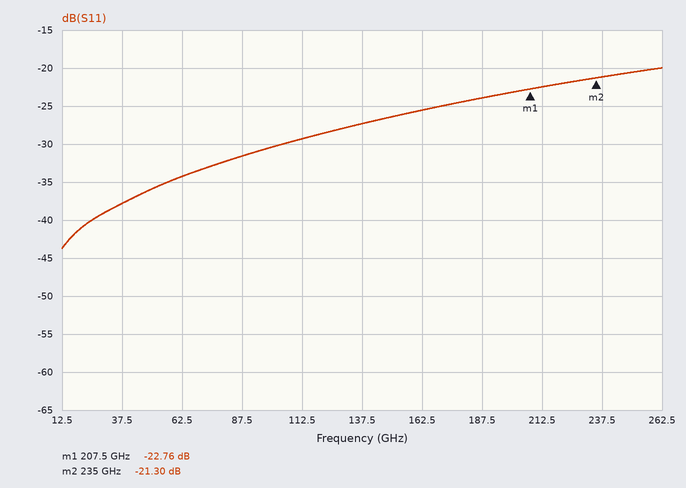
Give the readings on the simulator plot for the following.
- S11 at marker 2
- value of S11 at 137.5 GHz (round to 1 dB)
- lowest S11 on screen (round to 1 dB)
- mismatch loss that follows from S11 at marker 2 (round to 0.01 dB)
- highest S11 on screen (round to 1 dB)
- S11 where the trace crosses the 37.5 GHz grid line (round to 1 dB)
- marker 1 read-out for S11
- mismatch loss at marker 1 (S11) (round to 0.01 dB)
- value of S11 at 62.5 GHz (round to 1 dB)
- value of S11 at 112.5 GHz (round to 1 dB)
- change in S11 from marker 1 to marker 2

-21.30 dB
-27 dB
-44 dB
0.03 dB
-20 dB
-38 dB
-22.76 dB
0.02 dB
-34 dB
-29 dB
1.46 dB
